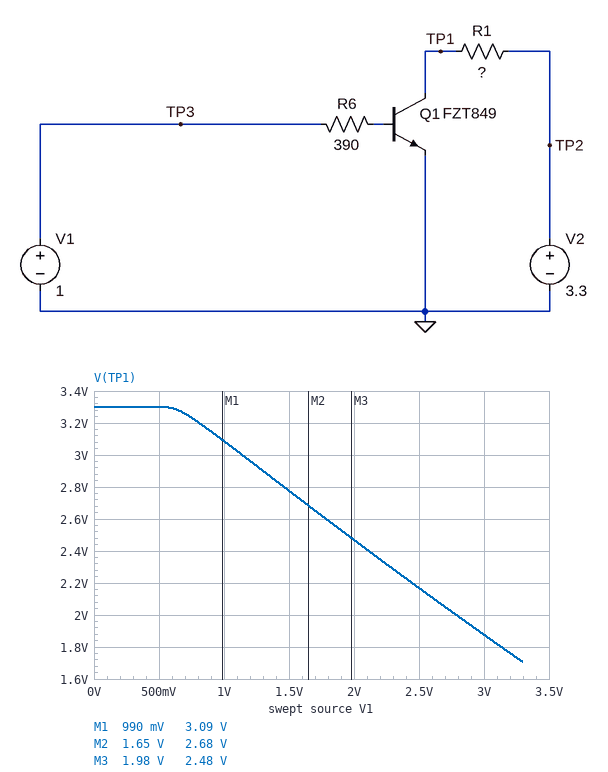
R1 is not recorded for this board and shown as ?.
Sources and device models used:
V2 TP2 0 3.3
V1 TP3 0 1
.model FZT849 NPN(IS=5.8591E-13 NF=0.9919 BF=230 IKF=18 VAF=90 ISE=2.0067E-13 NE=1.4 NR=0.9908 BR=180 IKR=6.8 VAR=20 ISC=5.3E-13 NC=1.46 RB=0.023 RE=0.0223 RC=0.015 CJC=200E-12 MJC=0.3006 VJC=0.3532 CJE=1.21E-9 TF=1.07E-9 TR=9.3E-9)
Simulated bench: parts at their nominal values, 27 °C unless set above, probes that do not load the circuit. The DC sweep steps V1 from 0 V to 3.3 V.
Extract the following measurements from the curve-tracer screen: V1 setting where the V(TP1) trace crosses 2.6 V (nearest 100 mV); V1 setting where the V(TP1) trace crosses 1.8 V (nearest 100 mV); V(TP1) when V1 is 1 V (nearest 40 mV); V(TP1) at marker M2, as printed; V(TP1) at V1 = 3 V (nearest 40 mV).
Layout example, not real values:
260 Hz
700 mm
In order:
1.8 V
3.1 V
3.08 V
2.68 V
1.88 V
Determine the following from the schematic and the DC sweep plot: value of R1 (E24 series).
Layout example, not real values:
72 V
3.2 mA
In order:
1.2 Ω
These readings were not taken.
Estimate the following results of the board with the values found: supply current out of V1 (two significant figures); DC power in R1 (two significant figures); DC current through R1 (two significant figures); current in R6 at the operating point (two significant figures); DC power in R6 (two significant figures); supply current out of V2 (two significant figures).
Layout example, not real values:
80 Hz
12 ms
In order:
810 µA
38 mW
180 mA
810 µA
260 µW
180 mA
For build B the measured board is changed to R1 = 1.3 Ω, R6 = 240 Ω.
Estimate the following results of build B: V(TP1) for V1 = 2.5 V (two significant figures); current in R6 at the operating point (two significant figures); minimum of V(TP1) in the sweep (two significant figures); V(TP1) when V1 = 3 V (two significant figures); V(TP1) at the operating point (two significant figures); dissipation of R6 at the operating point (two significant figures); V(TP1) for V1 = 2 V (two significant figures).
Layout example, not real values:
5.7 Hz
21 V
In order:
1.4 V
1.3 mA
660 mV
930 mV
2.9 V
380 µW
1.9 V
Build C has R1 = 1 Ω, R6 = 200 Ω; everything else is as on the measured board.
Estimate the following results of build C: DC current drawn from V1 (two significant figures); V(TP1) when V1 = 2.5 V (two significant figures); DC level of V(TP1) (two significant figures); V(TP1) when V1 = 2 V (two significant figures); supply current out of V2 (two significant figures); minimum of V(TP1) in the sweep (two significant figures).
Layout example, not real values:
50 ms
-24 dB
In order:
1.5 mA
1.6 V
3.0 V
2.0 V
320 mA
910 mV
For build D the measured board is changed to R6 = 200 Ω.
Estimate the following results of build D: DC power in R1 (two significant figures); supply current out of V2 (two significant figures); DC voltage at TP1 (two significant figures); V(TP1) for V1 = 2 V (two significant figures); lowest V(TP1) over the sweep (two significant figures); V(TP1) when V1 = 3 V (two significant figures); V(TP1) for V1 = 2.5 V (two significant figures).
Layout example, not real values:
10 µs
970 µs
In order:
130 mW
320 mA
2.9 V
1.8 V
440 mV
740 mV
1.2 V
